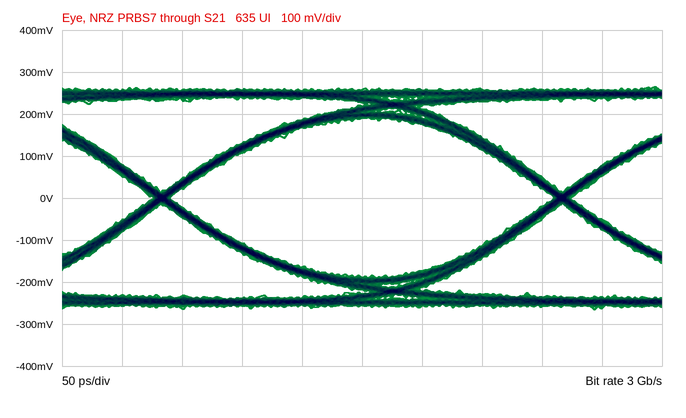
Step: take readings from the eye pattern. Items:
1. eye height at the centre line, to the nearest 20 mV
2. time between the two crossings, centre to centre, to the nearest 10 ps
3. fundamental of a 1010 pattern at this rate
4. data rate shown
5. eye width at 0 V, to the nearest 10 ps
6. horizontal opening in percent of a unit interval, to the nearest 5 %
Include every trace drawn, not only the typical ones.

380 mV
330 ps
1.5 GHz
3 Gb/s
320 ps
95 %
